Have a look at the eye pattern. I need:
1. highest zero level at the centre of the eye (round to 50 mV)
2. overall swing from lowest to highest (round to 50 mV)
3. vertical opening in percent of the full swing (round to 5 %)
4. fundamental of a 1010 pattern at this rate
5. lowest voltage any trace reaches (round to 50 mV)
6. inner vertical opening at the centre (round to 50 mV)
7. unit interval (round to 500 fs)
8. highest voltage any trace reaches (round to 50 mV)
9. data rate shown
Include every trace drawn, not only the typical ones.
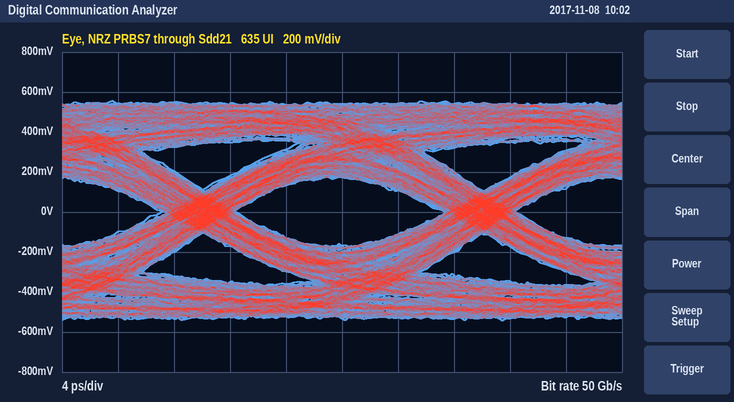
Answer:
-150 mV
1.10 V
30 %
25 GHz
-550 mV
350 mV
20.0 ps
550 mV
50 Gb/s
